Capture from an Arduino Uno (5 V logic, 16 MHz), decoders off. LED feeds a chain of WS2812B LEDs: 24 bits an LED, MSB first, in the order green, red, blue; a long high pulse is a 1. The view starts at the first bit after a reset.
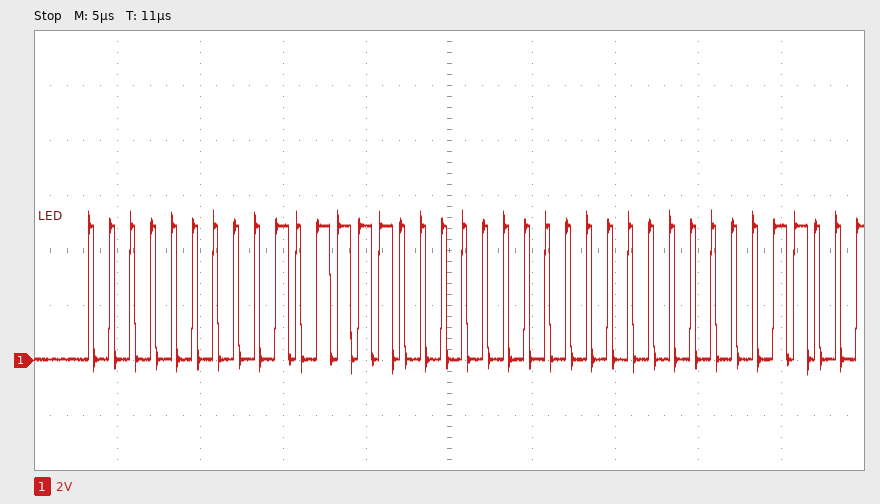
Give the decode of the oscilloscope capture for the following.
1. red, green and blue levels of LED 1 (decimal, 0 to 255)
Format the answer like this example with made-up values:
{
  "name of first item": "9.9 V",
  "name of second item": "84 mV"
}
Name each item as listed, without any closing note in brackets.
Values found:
{
  "red, green and blue levels of LED 1": "94, 0, 0"
}
